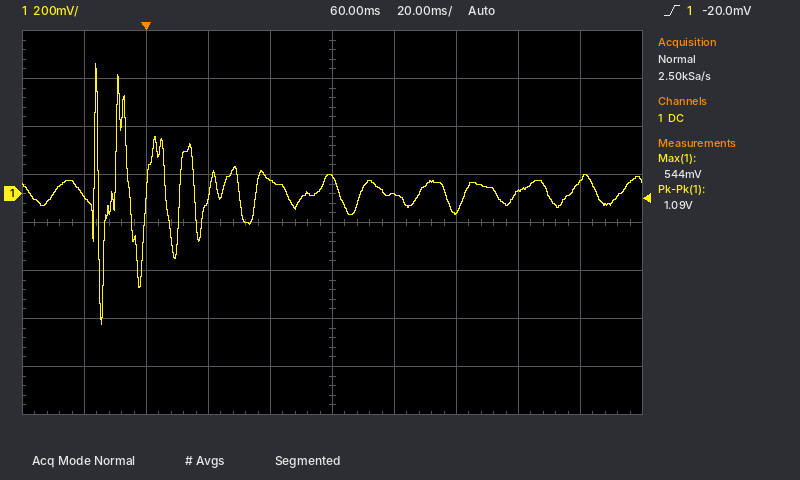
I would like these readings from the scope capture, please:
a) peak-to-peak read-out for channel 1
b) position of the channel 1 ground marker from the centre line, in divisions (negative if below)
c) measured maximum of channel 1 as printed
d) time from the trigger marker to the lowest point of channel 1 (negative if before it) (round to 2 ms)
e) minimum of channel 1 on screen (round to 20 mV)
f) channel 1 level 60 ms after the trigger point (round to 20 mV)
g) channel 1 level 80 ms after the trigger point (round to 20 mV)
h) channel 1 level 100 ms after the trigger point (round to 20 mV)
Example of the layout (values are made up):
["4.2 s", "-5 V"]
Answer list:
["1.09 V", "+0.6 div", "544 mV", "-14 ms", "-540 mV", "60 mV", "0 mV", "-80 mV"]
